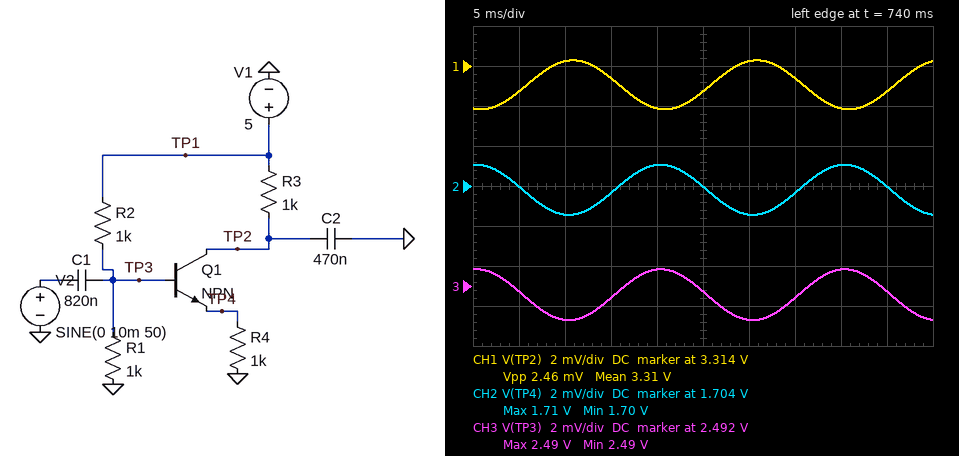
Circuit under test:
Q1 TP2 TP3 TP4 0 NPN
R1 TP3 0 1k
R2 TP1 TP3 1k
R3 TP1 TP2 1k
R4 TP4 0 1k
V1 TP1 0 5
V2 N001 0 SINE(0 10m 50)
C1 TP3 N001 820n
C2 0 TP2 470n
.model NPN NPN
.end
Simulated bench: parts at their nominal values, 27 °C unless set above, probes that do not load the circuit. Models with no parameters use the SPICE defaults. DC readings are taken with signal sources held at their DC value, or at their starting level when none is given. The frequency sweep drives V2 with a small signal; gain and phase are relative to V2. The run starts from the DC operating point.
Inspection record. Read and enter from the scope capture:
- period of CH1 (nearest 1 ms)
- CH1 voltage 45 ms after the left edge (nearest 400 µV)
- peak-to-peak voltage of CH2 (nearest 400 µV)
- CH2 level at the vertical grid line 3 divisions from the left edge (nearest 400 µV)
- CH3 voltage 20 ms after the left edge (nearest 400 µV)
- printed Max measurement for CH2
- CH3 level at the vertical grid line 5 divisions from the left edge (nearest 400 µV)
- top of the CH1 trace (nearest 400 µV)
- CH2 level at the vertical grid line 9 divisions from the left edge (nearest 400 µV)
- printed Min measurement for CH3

20 ms
3.3128 V
2.4 mV
1.7036 V
2.4928 V
1.71 V
2.4916 V
3.3144 V
1.7040 V
2.49 V
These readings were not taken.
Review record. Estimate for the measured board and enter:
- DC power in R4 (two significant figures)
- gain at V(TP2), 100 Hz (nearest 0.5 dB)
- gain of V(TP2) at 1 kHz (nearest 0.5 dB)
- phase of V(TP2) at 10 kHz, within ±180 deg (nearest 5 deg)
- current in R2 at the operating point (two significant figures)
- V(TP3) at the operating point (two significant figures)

2.9 mW
-12.5 dB
-10.5 dB
95 deg
2.5 mA
2.5 V
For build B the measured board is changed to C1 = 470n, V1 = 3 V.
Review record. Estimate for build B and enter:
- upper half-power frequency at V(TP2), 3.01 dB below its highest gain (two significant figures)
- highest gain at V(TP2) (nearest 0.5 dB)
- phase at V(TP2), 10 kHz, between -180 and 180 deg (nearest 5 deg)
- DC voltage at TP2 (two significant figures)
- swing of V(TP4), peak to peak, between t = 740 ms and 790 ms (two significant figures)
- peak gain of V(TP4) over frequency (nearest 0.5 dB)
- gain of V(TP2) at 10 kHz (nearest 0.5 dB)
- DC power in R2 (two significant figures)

1.2 kHz
-10.0 dB
95 deg
2.3 V
1.4 mV
-0.5 dB
-30.0 dB
2.3 mW
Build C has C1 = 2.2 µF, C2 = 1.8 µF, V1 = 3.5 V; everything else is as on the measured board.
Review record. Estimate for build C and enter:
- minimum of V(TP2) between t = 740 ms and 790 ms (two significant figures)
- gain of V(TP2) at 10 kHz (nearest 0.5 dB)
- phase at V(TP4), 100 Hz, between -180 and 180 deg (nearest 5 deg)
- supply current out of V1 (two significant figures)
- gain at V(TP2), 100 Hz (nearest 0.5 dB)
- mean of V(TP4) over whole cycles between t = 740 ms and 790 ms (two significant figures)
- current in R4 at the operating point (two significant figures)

2.5 V
-41.5 dB
55 deg
2.7 mA
-9.0 dB
970 mV
970 µA
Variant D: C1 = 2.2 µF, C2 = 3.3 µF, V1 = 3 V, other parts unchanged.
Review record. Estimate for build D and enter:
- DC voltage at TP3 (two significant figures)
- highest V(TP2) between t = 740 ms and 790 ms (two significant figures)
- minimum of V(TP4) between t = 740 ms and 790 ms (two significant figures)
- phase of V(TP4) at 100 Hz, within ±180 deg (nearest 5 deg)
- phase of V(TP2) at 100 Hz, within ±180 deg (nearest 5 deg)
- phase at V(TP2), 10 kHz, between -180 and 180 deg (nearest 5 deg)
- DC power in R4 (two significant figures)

1.5 V
2.3 V
730 mV
55 deg
170 deg
90 deg
530 µW
